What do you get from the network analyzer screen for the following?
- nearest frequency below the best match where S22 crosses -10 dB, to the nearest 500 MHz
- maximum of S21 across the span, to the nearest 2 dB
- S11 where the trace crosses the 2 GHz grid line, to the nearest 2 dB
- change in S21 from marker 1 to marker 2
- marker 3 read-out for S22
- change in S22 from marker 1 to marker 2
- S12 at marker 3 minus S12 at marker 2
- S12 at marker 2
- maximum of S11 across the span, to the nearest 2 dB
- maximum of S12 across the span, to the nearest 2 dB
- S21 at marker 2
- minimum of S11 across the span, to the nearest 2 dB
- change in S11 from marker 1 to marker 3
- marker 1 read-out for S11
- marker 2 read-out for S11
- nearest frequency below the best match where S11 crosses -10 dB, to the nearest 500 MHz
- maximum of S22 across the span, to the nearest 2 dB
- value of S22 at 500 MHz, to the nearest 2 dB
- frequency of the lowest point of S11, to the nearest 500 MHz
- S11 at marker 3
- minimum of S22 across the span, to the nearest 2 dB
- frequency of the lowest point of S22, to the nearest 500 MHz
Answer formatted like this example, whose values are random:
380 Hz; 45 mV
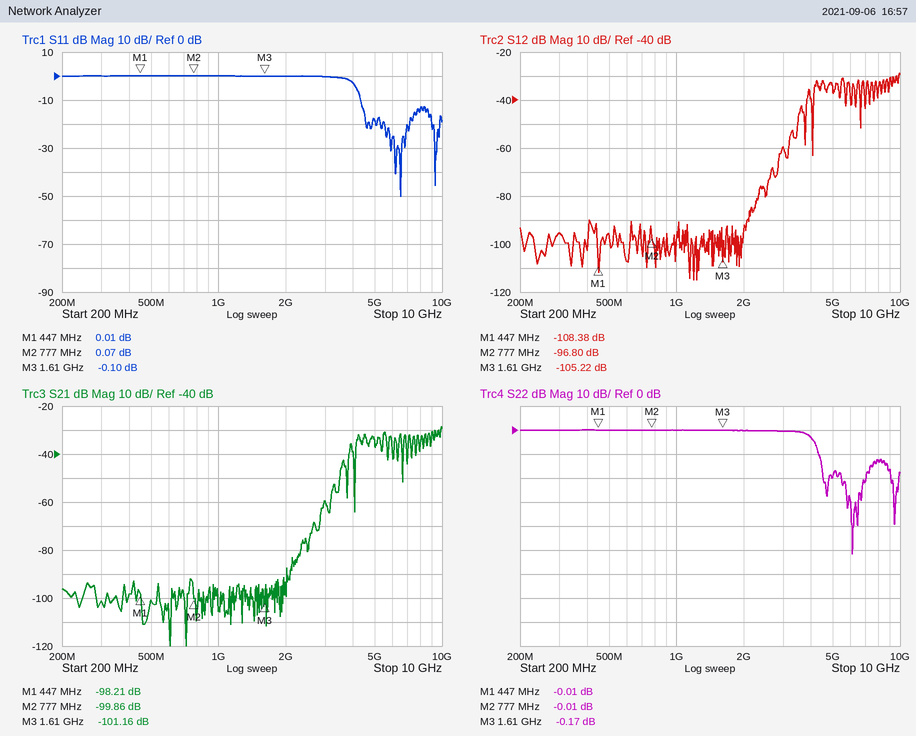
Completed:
4.5 GHz; -28 dB; 0 dB; -1.65 dB; -0.17 dB; 0.00 dB; -8.42 dB; -96.80 dB; 0 dB; -28 dB; -99.86 dB; -50 dB; -0.11 dB; 0.01 dB; 0.07 dB; 4.5 GHz; 0 dB; 0 dB; 6.5 GHz; -0.10 dB; -52 dB; 6.0 GHz
